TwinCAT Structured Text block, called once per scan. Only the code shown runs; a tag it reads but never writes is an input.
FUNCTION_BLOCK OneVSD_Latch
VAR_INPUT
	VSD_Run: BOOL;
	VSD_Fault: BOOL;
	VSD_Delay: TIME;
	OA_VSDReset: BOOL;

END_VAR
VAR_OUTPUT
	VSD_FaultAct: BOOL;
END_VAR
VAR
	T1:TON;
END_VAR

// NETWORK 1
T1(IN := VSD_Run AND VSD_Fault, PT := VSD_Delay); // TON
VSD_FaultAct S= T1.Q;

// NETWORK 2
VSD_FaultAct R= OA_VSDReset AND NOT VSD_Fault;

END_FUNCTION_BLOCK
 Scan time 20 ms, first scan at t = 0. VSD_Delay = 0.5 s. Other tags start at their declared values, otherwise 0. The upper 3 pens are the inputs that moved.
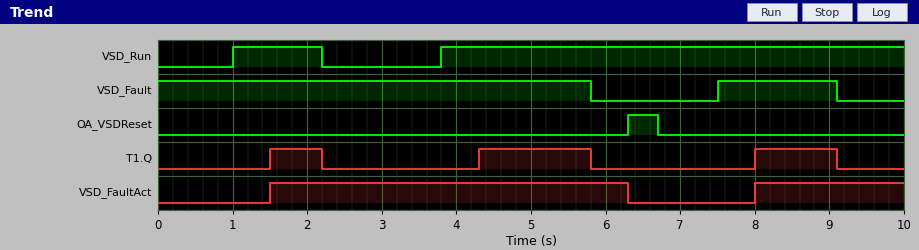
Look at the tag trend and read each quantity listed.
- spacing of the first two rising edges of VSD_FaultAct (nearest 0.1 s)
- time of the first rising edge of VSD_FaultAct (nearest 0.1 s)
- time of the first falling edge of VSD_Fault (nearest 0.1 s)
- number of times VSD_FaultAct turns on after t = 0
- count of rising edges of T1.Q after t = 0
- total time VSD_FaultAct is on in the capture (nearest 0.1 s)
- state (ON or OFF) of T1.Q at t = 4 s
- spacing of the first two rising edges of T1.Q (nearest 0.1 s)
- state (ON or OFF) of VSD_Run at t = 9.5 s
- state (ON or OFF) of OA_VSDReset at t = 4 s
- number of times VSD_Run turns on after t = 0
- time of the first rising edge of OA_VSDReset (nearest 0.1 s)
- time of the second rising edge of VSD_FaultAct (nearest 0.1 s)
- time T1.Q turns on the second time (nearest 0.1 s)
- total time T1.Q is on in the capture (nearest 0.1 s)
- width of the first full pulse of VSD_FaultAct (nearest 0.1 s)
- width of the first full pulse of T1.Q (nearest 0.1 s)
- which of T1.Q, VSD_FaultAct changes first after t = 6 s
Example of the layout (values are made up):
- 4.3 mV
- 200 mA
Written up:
- 6.5 s
- 1.5 s
- 5.8 s
- 2
- 3
- 6.8 s
- OFF
- 2.8 s
- ON
- OFF
- 2
- 6.3 s
- 8.0 s
- 4.3 s
- 3.3 s
- 4.8 s
- 0.7 s
- VSD_FaultAct
